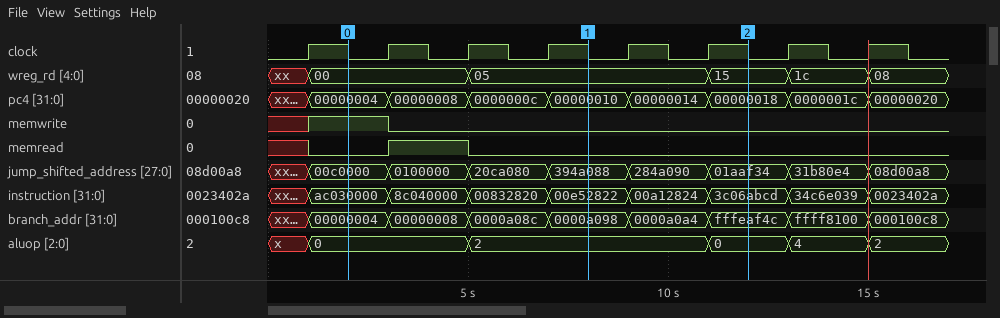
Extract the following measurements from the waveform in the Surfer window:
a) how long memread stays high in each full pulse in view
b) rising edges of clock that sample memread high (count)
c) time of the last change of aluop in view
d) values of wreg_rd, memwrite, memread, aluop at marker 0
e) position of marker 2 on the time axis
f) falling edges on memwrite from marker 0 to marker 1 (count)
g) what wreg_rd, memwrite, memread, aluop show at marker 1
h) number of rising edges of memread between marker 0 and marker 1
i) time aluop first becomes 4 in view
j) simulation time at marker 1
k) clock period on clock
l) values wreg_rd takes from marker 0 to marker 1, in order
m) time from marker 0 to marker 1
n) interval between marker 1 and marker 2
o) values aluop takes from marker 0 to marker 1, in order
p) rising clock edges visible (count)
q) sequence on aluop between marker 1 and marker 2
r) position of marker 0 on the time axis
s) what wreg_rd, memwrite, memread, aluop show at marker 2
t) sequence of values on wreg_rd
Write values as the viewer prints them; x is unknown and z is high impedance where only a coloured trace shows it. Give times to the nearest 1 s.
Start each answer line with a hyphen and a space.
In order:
- 2 s
- 1
- 15 s
- wreg_rd=00, memwrite=1, memread=0, aluop=0
- 12 s
- 1
- wreg_rd=05, memwrite=0, memread=0, aluop=2
- 1
- 13 s
- 8 s
- 2 s
- 00, 05
- 6 s
- 4 s
- 0, 2
- 8
- 2, 0
- 2 s
- wreg_rd=15, memwrite=0, memread=0, aluop=0
- xx, 00, 05, 15, 1c, 08
